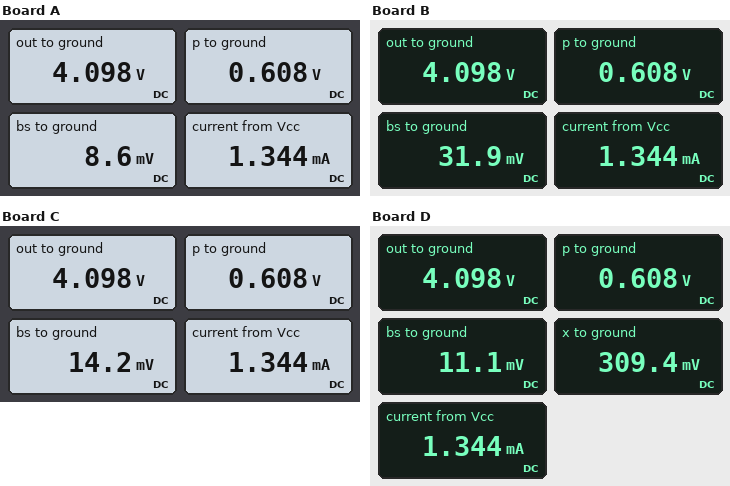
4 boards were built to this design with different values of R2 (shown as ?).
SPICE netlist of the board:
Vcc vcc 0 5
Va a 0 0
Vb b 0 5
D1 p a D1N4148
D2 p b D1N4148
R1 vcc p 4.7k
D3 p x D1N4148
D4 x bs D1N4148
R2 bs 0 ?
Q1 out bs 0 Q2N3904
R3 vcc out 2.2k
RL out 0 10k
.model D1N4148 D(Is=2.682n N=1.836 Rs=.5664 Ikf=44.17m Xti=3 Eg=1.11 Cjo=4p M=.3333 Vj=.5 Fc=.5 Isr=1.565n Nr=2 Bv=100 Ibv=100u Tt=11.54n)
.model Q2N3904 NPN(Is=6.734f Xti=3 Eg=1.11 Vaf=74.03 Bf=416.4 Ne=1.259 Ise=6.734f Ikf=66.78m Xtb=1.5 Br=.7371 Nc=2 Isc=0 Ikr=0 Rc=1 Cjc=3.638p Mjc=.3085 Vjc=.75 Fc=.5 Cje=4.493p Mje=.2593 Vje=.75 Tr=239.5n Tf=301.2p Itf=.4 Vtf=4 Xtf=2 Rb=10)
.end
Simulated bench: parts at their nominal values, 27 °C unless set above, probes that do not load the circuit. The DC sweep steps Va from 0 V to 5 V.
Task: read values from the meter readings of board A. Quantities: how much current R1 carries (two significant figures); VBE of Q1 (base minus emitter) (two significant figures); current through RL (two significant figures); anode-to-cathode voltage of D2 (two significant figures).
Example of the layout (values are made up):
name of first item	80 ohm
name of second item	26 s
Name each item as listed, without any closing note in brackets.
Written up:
how much current R1 carries	930 µA
VBE of Q1 (base minus emitter)	8.6 mV
current through RL	410 µA
anode-to-cathode voltage of D2	-4.4 V
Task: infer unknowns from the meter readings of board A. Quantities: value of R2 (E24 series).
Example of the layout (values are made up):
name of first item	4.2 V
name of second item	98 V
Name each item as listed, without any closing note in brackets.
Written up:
value of R2	4.7 kΩ
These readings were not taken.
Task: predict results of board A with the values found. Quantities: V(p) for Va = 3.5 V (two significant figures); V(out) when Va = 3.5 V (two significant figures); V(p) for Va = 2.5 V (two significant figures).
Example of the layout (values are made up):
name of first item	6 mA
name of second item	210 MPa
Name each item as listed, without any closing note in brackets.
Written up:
V(p) for Va = 3.5 V	1.9 V
V(out) when Va = 3.5 V	59 mV
V(p) for Va = 2.5 V	1.9 V
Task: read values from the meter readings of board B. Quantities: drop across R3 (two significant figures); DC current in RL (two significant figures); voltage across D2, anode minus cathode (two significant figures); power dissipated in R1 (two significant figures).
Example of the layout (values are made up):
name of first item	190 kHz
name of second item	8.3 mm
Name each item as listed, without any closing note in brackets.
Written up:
drop across R3	900 mV
DC current in RL	410 µA
voltage across D2, anode minus cathode	-4.4 V
power dissipated in R1	4.1 mW
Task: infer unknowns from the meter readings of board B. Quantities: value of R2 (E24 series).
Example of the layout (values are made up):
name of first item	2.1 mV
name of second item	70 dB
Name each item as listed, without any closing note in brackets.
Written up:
value of R2	22 kΩ
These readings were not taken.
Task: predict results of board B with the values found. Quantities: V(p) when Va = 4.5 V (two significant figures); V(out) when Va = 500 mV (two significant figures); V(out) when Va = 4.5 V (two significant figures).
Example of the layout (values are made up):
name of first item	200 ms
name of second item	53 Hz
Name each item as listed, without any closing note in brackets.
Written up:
V(p) when Va = 4.5 V	1.9 V
V(out) when Va = 500 mV	4.1 V
V(out) when Va = 4.5 V	55 mV
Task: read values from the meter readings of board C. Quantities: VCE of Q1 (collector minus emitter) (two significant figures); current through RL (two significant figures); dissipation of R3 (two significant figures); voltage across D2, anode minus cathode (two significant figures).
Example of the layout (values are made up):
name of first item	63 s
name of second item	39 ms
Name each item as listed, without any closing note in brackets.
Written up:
VCE of Q1 (collector minus emitter)	4.1 V
current through RL	410 µA
dissipation of R3	370 µW
voltage across D2, anode minus cathode	-4.4 V
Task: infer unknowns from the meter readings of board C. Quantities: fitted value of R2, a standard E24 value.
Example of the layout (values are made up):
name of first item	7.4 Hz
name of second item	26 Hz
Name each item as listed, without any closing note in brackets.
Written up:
fitted value of R2, a standard E24 value	8.2 kΩ
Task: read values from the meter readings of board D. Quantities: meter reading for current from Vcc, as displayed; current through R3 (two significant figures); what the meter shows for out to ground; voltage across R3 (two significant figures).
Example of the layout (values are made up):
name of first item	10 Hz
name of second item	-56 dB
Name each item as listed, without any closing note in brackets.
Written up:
meter reading for current from Vcc, as displayed	1.344 mA
current through R3	410 µA
what the meter shows for out to ground	4.098 V
voltage across R3	900 mV
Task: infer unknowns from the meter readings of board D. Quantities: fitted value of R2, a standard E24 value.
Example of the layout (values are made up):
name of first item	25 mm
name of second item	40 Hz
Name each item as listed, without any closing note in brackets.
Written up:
fitted value of R2, a standard E24 value	6.2 kΩ
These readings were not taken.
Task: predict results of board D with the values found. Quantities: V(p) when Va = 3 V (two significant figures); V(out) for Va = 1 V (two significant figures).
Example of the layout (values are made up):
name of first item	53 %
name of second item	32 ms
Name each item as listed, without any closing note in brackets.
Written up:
V(p) when Va = 3 V	1.9 V
V(out) for Va = 1 V	4.0 V
